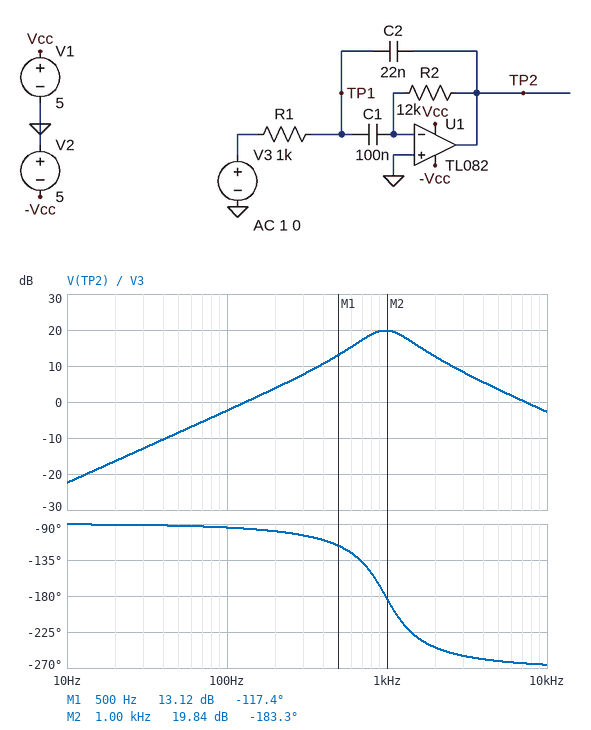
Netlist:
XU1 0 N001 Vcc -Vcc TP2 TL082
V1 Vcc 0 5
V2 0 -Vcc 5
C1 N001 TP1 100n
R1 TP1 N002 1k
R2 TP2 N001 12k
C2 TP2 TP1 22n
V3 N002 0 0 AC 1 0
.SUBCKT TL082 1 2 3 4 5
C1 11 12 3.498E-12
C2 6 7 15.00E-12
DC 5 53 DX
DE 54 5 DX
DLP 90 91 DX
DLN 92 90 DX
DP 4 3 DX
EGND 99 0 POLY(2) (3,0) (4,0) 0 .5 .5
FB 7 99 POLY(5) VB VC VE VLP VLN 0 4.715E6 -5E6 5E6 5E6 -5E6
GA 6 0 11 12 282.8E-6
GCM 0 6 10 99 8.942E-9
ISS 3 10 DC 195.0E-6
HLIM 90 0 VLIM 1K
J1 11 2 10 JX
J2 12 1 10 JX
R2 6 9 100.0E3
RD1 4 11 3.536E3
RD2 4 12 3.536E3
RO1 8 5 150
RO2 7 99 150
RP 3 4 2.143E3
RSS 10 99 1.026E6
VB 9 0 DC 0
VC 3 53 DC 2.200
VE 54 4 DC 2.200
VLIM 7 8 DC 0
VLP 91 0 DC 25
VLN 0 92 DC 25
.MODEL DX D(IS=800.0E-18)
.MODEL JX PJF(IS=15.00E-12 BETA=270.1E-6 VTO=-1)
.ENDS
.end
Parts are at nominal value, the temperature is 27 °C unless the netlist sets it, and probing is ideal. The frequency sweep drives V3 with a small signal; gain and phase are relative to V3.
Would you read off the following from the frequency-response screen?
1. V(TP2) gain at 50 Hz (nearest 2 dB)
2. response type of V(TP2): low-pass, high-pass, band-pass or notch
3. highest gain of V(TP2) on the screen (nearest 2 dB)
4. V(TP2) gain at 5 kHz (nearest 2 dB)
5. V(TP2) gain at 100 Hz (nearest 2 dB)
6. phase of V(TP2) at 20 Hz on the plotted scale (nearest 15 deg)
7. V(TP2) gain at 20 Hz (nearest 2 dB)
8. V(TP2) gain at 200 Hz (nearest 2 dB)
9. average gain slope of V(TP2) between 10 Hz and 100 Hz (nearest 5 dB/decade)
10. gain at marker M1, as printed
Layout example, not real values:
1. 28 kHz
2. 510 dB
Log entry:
1. -8 dB
2. band-pass
3. 20 dB
4. 4 dB
5. -2 dB
6. -90 deg
7. -16 dB
8. 4 dB
9. 20 dB/decade
10. 13.12 dB
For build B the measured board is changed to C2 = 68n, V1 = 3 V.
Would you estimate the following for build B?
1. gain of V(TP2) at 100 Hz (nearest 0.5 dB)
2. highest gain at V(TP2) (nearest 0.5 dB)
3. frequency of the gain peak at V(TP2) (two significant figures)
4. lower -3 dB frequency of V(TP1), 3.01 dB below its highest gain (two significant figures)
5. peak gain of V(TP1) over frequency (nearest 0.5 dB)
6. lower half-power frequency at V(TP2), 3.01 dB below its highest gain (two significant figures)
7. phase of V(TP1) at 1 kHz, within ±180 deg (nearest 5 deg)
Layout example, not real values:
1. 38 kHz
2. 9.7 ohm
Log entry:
1. -2.0 dB
2. 17.0 dB
3. 560 Hz
4. 290 Hz
5. 5.0 dB
6. 420 Hz
7. -155 deg
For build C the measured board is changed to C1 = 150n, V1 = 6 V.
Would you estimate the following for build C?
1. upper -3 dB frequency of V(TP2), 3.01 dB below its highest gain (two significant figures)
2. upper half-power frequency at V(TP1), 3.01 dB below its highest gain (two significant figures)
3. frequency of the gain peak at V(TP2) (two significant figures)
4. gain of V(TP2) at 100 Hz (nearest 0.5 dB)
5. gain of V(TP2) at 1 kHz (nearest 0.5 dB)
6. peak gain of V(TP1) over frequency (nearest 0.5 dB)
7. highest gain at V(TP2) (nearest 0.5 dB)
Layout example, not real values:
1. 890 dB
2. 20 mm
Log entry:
1. 1.2 kHz
2. 950 Hz
3. 800 Hz
4. 1.0 dB
5. 19.5 dB
6. 2.0 dB
7. 20.5 dB
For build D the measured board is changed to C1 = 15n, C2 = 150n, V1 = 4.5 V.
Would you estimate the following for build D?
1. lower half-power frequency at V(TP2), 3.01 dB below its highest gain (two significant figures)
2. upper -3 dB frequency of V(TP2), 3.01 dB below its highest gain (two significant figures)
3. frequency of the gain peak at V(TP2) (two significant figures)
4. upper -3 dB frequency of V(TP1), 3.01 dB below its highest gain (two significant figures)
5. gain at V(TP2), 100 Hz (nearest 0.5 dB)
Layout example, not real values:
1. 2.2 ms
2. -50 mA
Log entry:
1. 600 Hz
2. 1.6 kHz
3. 970 Hz
4. 1.1 kHz
5. -19.0 dB
